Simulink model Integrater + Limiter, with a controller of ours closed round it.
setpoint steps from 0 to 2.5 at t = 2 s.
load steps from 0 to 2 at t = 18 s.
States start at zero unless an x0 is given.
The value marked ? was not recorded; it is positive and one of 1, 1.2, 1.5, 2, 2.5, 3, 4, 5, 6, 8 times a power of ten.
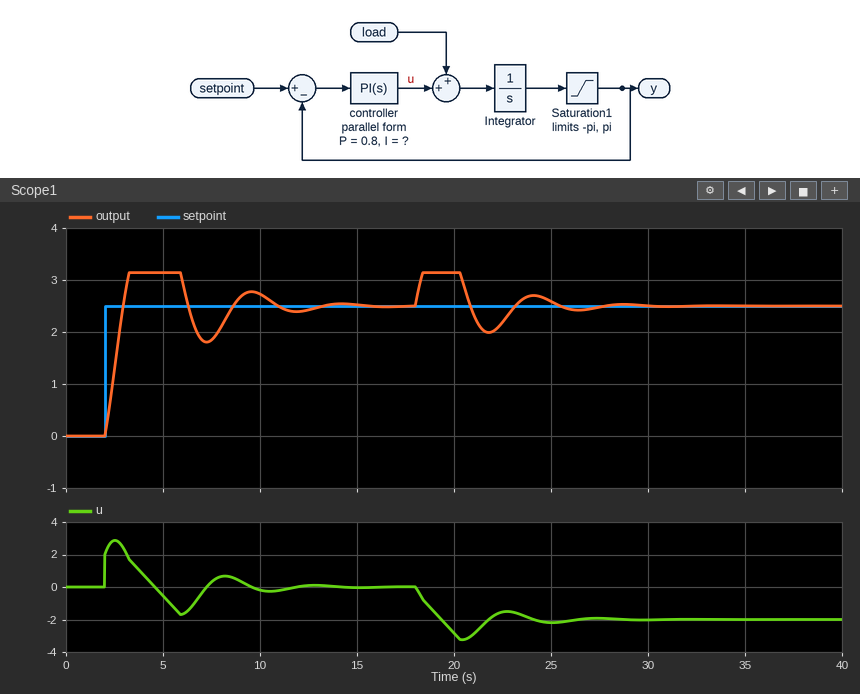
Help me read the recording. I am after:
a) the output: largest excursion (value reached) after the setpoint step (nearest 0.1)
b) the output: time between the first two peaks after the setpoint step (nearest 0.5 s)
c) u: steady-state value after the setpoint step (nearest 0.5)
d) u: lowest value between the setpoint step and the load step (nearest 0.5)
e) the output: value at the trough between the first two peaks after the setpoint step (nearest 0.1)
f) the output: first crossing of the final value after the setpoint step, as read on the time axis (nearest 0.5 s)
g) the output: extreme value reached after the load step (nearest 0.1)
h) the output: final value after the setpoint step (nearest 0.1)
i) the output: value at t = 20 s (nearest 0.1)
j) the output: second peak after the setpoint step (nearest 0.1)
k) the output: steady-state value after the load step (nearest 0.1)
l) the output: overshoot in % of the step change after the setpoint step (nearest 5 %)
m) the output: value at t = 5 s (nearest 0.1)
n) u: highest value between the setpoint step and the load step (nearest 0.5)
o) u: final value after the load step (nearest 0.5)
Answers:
3.1
5.0 s
0.0
-1.5
1.8
3.0 s
3.1
2.5
3.1
2.8
2.5
25 %
3.1
3.0
-2.0
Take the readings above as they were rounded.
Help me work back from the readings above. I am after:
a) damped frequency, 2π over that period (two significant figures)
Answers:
1.3 rad/s
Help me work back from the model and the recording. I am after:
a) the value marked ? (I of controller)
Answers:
2
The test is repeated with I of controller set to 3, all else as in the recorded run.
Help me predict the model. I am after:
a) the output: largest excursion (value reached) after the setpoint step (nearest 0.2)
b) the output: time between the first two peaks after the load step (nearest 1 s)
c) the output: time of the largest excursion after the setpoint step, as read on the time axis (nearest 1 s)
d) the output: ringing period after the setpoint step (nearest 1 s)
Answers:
3.2
4 s
3 s
4 s
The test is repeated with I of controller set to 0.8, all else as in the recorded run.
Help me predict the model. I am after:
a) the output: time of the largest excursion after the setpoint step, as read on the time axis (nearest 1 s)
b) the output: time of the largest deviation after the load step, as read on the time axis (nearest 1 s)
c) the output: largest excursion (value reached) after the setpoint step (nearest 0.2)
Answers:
4 s
18 s
3.2
